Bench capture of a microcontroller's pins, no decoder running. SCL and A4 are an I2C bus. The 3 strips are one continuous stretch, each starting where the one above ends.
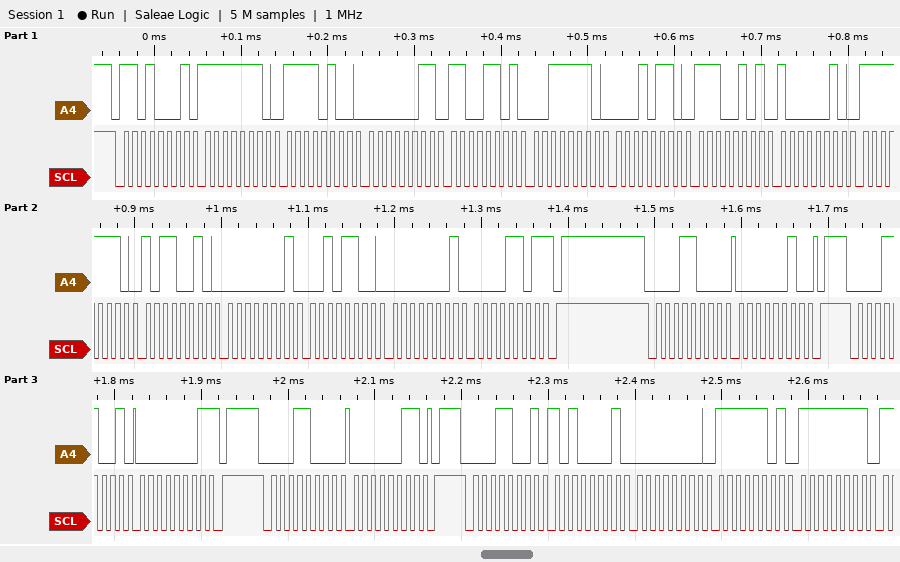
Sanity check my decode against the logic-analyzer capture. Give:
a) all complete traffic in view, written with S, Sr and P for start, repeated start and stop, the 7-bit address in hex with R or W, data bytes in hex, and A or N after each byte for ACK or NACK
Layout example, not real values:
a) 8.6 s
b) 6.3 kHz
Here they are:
a) S 68R A FE A F4 A 03 A CD A 3E A 16 A E5 A 82 A FE A B2 A 01 A 2C A 01 A 0D N P S 0CW A 02 A P S 0CR A 01 N P S 0CW A 03 A P S 0CR A A1 A 00 A FD A FF A
